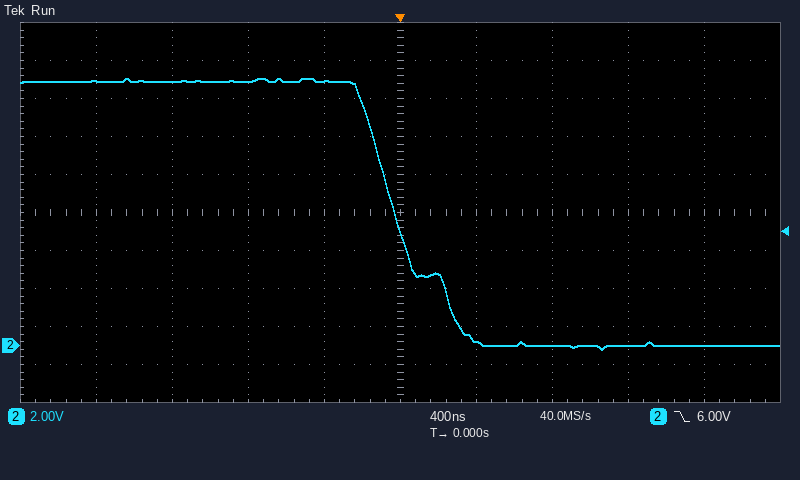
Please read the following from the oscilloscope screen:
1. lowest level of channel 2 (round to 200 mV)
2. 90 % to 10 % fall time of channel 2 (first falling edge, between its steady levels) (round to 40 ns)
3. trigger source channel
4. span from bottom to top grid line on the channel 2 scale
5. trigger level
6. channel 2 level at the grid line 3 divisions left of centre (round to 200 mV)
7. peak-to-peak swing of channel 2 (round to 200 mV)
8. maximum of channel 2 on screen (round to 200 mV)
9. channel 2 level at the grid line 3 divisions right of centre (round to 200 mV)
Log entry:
-200 mV
480 ns
channel 2
20 V
6.00 V
13.8 V
14.2 V
14.0 V
0.0 V
